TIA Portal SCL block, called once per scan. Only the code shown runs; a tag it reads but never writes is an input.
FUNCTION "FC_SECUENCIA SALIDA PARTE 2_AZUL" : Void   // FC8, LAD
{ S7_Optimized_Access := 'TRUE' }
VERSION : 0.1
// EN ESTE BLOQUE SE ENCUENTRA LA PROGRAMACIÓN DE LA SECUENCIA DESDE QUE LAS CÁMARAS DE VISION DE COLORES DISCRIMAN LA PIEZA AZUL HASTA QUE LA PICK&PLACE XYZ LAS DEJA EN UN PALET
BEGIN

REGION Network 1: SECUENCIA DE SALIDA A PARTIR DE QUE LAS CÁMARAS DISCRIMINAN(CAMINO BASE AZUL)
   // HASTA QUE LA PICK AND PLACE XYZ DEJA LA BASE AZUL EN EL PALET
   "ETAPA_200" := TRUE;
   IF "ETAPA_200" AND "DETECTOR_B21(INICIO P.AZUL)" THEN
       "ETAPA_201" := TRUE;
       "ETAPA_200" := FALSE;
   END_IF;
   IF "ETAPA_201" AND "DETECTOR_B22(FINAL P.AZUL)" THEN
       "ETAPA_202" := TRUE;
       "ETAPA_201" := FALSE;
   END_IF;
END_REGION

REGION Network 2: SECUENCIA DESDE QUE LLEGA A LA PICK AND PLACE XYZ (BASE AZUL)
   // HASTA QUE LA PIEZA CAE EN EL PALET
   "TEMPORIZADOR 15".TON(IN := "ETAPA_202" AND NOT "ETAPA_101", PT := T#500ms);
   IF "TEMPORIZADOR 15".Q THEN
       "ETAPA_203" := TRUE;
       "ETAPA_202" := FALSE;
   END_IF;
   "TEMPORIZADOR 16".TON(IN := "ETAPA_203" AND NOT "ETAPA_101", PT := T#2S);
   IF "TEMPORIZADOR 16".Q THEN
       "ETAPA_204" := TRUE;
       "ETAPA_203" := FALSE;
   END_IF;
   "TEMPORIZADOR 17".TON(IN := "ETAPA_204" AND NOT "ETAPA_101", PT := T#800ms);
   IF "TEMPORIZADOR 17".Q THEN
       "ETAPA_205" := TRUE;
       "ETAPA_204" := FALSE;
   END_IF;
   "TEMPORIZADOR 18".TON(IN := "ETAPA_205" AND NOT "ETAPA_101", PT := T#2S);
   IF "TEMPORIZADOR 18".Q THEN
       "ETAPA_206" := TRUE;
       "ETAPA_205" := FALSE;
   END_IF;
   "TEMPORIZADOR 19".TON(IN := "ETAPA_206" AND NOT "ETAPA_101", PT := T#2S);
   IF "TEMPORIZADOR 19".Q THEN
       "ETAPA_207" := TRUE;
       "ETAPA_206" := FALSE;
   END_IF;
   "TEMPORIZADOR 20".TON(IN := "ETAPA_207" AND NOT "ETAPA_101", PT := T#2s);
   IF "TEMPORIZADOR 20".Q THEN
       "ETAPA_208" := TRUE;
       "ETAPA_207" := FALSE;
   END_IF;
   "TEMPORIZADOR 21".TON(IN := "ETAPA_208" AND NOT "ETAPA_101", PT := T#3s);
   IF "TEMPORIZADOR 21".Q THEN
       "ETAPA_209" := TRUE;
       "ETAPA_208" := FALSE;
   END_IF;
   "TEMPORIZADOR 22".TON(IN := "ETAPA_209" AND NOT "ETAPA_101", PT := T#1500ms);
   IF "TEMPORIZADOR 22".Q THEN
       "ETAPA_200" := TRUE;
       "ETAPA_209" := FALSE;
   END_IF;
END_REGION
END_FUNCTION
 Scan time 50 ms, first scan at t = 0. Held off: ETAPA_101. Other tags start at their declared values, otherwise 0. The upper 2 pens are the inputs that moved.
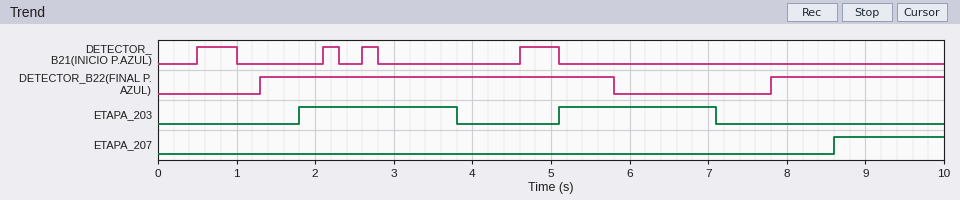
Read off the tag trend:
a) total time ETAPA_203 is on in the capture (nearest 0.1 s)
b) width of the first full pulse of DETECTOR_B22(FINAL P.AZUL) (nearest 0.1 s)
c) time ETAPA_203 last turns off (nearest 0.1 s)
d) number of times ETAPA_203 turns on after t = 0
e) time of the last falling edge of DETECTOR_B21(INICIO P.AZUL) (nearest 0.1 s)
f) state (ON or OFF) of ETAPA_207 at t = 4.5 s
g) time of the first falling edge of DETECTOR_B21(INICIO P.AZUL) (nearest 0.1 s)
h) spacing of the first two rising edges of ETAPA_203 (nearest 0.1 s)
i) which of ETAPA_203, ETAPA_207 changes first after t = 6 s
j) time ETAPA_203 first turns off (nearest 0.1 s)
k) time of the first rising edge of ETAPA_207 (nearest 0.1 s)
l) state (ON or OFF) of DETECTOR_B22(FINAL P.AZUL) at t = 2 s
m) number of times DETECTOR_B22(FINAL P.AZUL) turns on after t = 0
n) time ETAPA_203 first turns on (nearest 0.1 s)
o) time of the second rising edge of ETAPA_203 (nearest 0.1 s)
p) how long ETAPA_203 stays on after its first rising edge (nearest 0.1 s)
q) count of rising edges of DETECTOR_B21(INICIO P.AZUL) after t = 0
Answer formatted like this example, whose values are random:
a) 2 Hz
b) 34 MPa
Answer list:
a) 4.0 s
b) 4.5 s
c) 7.1 s
d) 2
e) 5.1 s
f) OFF
g) 1.0 s
h) 3.3 s
i) ETAPA_203
j) 3.8 s
k) 8.6 s
l) ON
m) 2
n) 1.8 s
o) 5.1 s
p) 2.0 s
q) 4
